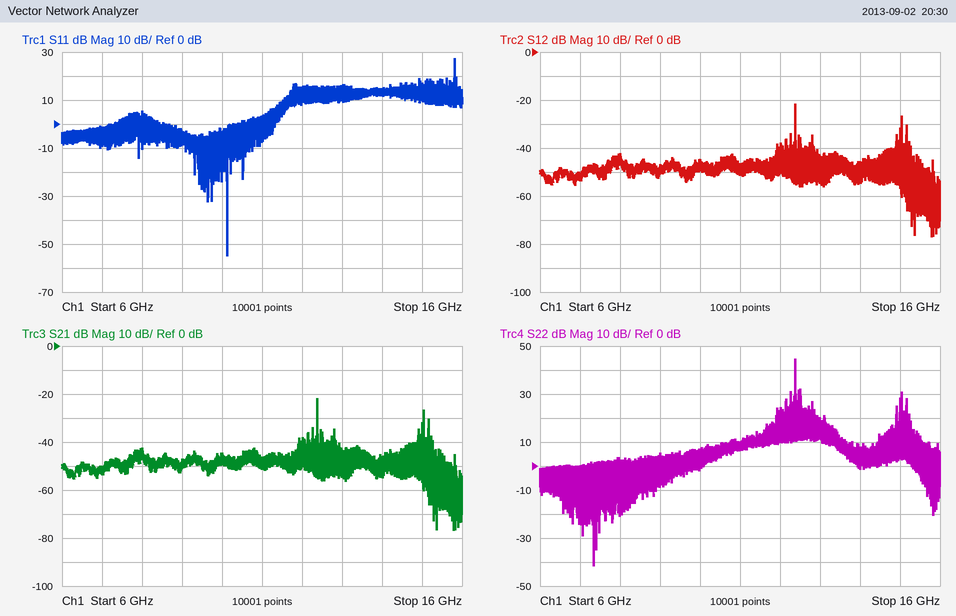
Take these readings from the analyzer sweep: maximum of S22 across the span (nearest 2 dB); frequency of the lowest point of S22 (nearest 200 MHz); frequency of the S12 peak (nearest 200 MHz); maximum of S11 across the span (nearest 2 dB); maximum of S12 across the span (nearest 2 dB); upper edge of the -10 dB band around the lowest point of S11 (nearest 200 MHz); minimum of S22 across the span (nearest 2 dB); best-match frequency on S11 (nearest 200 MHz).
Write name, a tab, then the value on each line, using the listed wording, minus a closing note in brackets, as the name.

maximum of S22 across the span	44 dB
frequency of the lowest point of S22	7.4 GHz
frequency of the S12 peak	12.4 GHz
maximum of S11 across the span	28 dB
maximum of S12 across the span	-22 dB
upper edge of the -10 dB band around the lowest point of S11	10.2 GHz
minimum of S22 across the span	-42 dB
best-match frequency on S11	10.2 GHz
